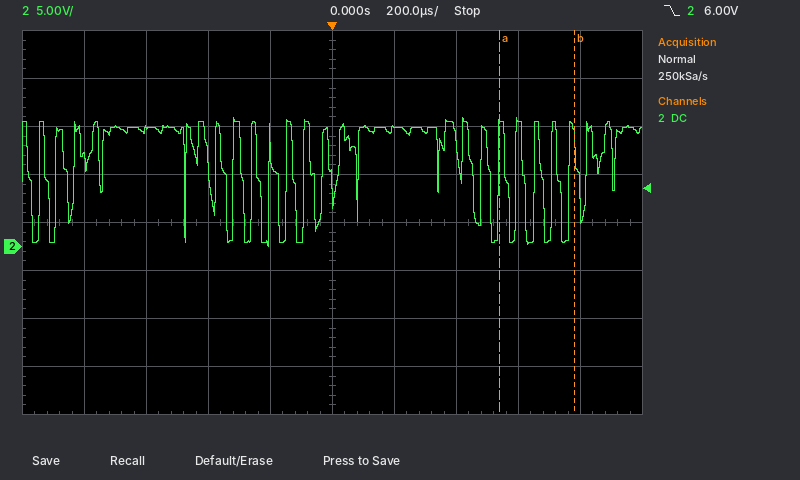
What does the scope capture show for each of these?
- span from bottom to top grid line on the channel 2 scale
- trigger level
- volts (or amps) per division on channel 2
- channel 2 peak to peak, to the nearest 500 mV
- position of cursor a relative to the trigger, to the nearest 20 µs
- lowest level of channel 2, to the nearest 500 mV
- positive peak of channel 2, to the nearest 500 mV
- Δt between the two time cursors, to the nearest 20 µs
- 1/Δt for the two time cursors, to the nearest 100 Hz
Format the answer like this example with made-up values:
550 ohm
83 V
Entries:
40 V
6.00 V
5 V
13.5 V
+540 µs
0.0 V
13.5 V
240 µs
4.2 kHz
